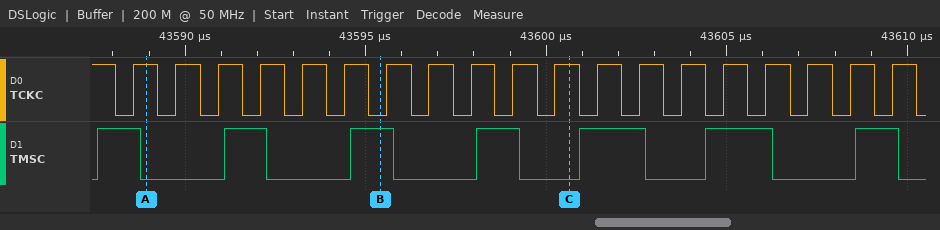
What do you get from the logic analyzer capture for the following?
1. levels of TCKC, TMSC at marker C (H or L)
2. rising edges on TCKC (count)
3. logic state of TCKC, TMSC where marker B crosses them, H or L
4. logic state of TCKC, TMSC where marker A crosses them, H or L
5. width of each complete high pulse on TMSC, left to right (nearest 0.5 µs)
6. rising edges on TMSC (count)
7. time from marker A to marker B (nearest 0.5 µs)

TCKC=H, TMSC=L
19
TCKC=L, TMSC=H
TCKC=H, TMSC=L
1 µs, 1 µs, 1 µs, 1 µs, 2 µs, 2 µs, 1 µs
7
6.5 µs
